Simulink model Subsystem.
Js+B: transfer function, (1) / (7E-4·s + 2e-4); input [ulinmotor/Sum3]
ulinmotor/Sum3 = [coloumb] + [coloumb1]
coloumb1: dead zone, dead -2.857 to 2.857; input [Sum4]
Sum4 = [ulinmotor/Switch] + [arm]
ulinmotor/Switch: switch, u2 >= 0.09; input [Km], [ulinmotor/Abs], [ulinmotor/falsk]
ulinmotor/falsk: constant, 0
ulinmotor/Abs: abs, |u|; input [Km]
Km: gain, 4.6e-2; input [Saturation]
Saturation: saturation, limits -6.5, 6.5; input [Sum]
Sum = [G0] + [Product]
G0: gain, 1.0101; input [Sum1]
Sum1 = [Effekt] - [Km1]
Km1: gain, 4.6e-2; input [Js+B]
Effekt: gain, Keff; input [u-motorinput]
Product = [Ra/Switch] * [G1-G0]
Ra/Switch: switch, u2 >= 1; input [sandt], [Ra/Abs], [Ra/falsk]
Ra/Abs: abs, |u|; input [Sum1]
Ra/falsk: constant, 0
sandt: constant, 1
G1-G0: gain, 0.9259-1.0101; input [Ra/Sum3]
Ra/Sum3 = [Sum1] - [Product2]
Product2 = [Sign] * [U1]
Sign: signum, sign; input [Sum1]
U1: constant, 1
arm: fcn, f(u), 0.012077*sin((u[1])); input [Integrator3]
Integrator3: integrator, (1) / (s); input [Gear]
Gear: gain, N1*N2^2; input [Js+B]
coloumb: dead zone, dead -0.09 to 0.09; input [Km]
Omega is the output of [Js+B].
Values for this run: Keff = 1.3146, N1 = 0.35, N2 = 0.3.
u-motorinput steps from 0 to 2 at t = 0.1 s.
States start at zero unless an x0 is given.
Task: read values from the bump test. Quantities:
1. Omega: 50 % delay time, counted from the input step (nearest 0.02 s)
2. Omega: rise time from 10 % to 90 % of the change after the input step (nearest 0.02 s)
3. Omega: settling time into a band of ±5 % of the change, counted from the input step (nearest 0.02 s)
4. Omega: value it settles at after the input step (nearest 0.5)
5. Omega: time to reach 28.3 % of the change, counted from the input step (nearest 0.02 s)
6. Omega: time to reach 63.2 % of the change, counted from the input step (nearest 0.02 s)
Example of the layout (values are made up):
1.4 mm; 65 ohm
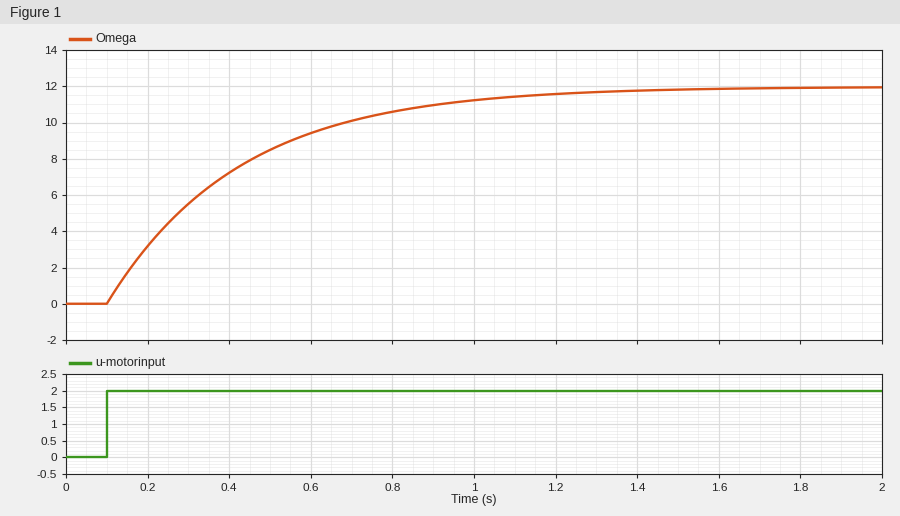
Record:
0.22 s; 0.72 s; 0.98 s; 12.0; 0.10 s; 0.32 s
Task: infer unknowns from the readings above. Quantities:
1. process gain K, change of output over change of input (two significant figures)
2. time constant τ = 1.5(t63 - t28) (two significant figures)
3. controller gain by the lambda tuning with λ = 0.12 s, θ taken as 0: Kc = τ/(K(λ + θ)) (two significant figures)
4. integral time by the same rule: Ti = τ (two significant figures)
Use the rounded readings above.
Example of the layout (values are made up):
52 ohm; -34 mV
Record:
6.0; 0.33 s; 0.46; 0.33 s
